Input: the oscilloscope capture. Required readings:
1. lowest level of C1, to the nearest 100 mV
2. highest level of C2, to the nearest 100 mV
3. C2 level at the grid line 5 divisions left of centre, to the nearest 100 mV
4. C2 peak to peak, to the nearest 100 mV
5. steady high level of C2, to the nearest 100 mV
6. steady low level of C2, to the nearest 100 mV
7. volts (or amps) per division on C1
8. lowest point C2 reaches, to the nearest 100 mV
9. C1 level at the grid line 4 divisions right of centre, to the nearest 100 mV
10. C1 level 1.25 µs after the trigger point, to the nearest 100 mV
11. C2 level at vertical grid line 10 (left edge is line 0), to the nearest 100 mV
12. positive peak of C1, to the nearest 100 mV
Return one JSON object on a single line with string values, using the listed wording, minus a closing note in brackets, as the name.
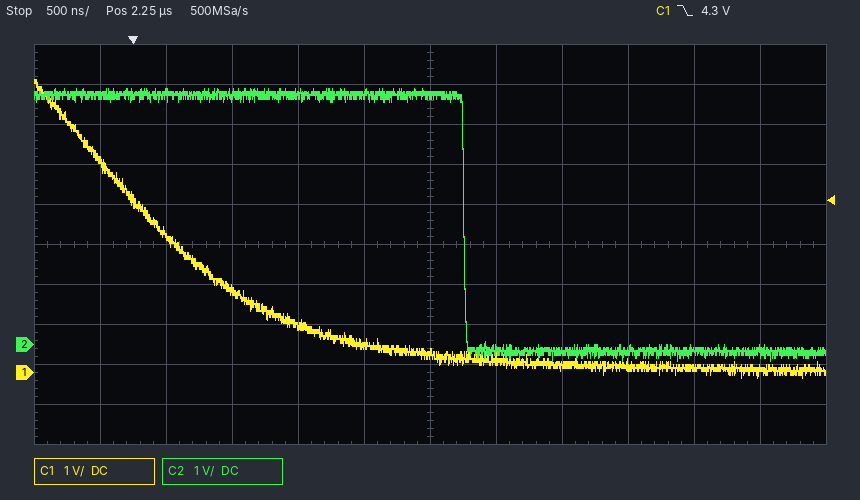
{"lowest level of C1, to the nearest 100 mV": "-100 mV", "highest level of C2, to the nearest 100 mV": "6.4 V", "C2 level at the grid line 5 divisions left of centre, to the nearest 100 mV": "6.2 V", "C2 peak to peak, to the nearest 100 mV": "6.8 V", "steady high level of C2, to the nearest 100 mV": "6.2 V", "steady low level of C2, to the nearest 100 mV": "-200 mV", "volts (or amps) per division on C1": "1 V", "lowest point C2 reaches, to the nearest 100 mV": "-400 mV", "C1 level at the grid line 4 divisions right of centre, to the nearest 100 mV": "100 mV", "C1 level 1.25 µs after the trigger point, to the nearest 100 mV": "1.2 V", "C2 level at vertical grid line 10 (left edge is line 0), to the nearest 100 mV": "-200 mV", "positive peak of C1, to the nearest 100 mV": "7.3 V"}
